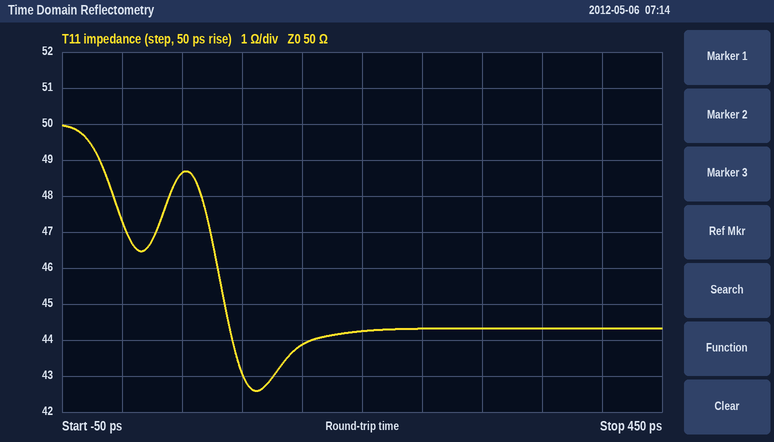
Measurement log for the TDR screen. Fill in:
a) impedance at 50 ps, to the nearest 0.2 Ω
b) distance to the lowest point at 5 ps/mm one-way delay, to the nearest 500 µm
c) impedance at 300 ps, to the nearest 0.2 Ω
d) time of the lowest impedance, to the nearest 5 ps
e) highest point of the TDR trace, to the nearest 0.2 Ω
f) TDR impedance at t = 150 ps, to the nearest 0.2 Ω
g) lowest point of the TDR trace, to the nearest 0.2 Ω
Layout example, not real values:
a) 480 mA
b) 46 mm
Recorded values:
a) 48.6 Ω
b) 11.0 mm
c) 44.4 Ω
d) 110 ps
e) 50.0 Ω
f) 43.8 Ω
g) 42.6 Ω
